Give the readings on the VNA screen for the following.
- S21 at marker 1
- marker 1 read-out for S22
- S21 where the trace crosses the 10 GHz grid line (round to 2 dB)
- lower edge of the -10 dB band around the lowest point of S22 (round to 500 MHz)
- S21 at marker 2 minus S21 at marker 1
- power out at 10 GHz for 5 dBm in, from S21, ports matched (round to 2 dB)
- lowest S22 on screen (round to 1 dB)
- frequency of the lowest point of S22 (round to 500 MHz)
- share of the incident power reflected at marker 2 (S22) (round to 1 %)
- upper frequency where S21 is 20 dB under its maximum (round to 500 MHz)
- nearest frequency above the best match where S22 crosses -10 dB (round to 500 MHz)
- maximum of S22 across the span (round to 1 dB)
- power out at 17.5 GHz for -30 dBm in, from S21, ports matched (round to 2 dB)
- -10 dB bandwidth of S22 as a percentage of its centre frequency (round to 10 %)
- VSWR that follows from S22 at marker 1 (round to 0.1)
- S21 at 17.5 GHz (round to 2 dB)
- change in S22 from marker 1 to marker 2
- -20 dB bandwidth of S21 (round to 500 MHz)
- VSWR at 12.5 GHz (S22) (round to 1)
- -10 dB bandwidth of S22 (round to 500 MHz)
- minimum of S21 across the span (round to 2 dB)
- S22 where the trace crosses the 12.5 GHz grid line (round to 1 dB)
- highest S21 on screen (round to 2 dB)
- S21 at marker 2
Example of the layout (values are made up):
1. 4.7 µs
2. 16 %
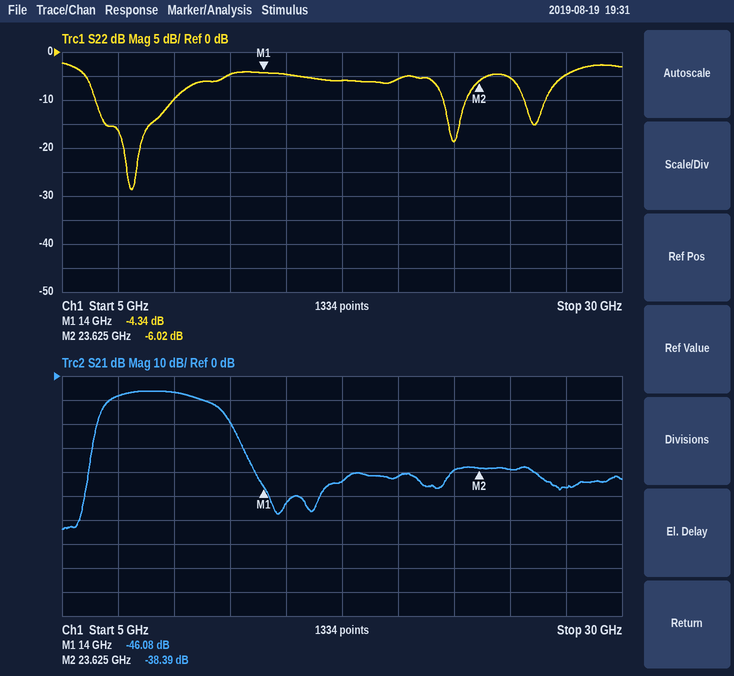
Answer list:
1. -46.08 dB
2. -4.34 dB
3. -6 dB
4. 6.5 GHz
5. 7.69 dB
6. -2 dBm
7. -29 dB
8. 8.0 GHz
9. 25 %
10. 13.0 GHz
11. 10.0 GHz
12. -2 dB
13. -74 dBm
14. 40 %
15. 4.1
16. -44 dB
17. -1.68 dB
18. 6.5 GHz
19. 4
20. 3.5 GHz
21. -64 dB
22. -5 dB
23. -6 dB
24. -38.39 dB
